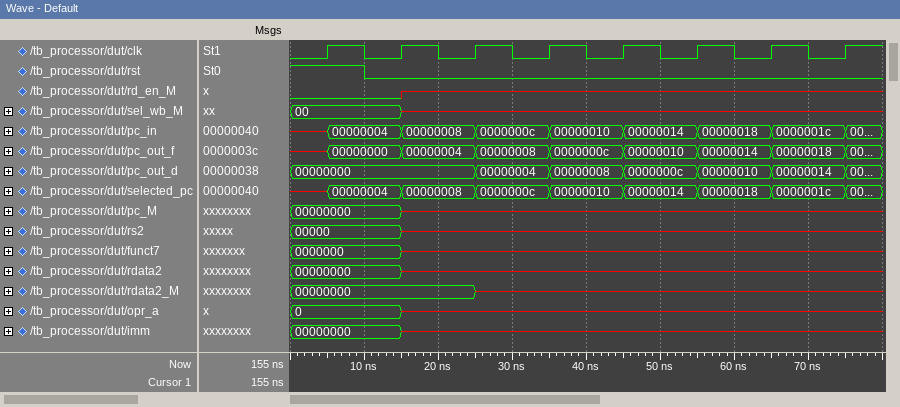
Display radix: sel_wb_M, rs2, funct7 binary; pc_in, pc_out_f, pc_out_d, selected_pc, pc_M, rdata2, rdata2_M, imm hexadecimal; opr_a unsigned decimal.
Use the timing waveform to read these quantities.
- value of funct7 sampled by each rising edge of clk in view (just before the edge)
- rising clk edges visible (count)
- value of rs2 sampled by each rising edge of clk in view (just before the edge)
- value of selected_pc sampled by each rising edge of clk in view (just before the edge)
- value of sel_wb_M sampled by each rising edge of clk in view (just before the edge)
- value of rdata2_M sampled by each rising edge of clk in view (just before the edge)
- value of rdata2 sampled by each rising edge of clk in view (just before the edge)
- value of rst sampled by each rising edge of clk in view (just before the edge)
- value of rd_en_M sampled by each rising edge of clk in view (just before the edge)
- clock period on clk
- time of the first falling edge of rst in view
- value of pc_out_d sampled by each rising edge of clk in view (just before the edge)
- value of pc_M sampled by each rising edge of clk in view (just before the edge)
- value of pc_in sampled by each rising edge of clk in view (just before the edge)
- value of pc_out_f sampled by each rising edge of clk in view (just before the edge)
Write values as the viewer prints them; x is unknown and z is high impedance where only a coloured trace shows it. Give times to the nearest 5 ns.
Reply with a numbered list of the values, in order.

1. 0000000, 0000000, x, x, x, x, x, x
2. 8
3. 00000, 00000, x, x, x, x, x, x
4. x, 00000004, 00000008, 0000000c, 00000010, 00000014, 00000018, 0000001c
5. 00, 00, x, x, x, x, x, x
6. 00000000, 00000000, 00000000, x, x, x, x, x
7. 00000000, 00000000, x, x, x, x, x, x
8. 1 0 0 0 0 0 0 0
9. 0 0 x x x x x x
10. 10 ns
11. 10 ns
12. 00000000, 00000000, 00000000, 00000004, 00000008, 0000000c, 00000010, 00000014
13. 00000000, 00000000, x, x, x, x, x, x
14. x, 00000004, 00000008, 0000000c, 00000010, 00000014, 00000018, 0000001c
15. x, 00000000, 00000004, 00000008, 0000000c, 00000010, 00000014, 00000018
